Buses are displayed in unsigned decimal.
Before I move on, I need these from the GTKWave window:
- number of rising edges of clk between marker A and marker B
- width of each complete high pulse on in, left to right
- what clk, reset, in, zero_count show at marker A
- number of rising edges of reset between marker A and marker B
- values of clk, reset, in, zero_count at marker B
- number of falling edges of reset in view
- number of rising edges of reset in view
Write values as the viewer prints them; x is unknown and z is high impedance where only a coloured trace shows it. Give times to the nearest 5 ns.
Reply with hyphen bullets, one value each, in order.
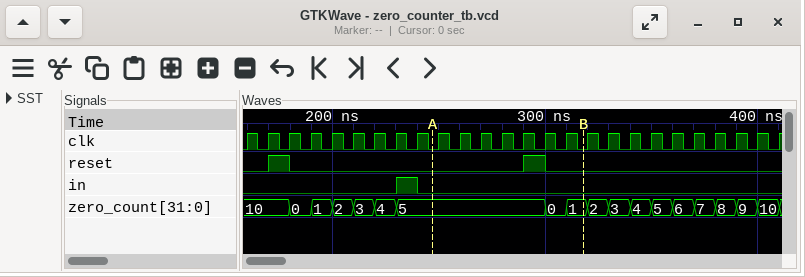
- 7
- 10 ns
- clk=0, reset=0, in=0, zero_count=5
- 1
- clk=0, reset=0, in=0, zero_count=1
- 2
- 2
